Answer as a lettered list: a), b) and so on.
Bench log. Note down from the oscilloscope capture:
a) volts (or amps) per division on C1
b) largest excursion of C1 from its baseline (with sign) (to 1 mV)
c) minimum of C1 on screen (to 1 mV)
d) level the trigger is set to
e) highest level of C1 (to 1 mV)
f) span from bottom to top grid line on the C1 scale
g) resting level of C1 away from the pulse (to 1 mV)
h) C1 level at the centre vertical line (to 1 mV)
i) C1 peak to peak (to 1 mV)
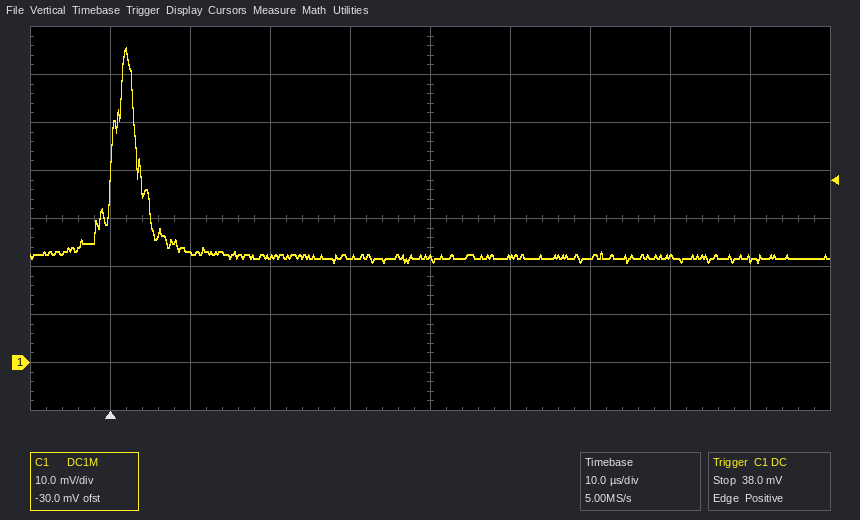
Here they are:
a) 10 mV
b) +44 mV
c) 21 mV
d) 38.0 mV
e) 66 mV
f) 80 mV
g) 22 mV
h) 22 mV
i) 45 mV
